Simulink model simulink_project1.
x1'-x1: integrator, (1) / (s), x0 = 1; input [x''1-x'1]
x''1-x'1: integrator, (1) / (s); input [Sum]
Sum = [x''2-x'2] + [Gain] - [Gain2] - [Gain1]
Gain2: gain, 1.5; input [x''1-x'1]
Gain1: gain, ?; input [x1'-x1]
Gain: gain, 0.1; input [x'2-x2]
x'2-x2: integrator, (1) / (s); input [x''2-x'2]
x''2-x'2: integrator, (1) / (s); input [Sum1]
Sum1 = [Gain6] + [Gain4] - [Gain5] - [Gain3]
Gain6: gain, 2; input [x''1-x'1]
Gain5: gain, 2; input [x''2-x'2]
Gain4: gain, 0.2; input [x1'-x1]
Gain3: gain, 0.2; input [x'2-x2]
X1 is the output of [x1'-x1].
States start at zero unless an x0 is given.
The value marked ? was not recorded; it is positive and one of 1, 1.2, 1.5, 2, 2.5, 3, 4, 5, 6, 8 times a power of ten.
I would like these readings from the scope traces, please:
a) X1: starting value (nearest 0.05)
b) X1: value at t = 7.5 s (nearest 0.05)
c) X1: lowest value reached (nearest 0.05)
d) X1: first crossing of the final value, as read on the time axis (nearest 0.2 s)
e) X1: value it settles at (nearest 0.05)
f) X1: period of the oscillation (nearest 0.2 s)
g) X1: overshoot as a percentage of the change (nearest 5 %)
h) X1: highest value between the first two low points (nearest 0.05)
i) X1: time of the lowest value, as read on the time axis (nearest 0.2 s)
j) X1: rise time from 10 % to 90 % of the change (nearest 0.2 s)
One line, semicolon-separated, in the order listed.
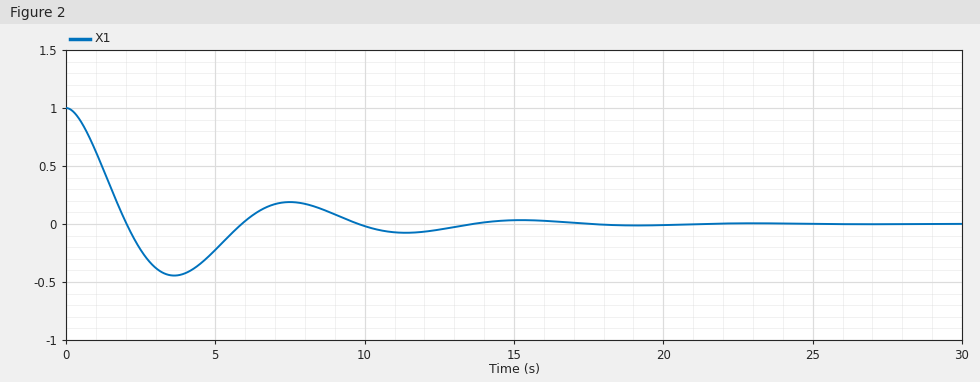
1.00; 0.20; -0.45; 2.0 s; 0.00; 7.8 s; 45 %; 0.20; 3.6 s; 1.4 s
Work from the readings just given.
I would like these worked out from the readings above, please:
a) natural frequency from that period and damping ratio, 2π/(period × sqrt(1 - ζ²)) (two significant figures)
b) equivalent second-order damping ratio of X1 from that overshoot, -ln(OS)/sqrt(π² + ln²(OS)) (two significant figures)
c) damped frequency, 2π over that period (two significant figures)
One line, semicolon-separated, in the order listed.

0.83 rad/s; 0.25; 0.81 rad/s
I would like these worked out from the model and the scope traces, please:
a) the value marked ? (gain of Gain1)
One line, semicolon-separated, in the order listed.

1.2
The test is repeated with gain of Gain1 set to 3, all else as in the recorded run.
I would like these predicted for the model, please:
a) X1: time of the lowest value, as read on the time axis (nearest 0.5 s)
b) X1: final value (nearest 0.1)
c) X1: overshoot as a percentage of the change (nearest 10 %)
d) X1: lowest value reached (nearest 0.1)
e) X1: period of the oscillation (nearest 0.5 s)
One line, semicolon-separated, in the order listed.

2.0 s; 0.0; 50 %; -0.5; 4.5 s
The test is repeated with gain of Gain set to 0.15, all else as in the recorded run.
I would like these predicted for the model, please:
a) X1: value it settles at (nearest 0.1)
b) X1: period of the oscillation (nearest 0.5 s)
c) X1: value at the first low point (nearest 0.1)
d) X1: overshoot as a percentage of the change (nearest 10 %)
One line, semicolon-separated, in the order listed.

0.0; 8.0 s; -0.5; 50 %
